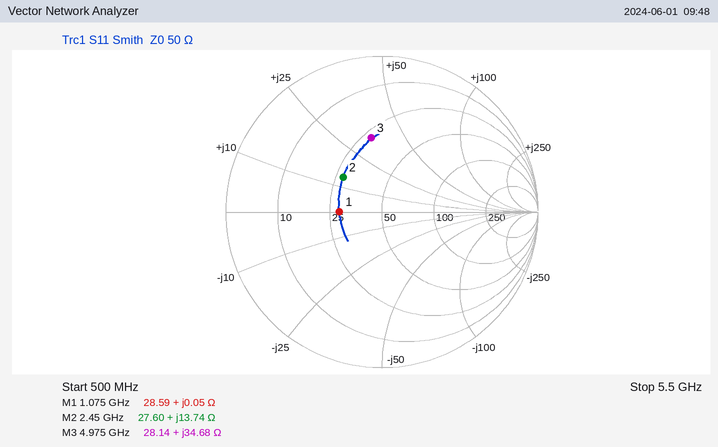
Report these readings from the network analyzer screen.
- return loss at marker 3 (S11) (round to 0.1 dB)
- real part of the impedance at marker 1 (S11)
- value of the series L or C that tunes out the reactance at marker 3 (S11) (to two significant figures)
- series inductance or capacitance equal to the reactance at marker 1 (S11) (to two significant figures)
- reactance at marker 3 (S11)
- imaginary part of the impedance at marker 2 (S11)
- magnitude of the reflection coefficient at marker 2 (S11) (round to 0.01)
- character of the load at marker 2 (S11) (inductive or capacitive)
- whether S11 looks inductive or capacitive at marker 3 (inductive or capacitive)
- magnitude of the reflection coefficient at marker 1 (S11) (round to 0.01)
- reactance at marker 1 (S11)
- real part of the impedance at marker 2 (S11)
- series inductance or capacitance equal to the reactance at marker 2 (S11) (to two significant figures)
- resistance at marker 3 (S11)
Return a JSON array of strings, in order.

["6.4 dB", "28.59 Ω", "920 fF", "7.4 pH", "+34.68 Ω", "+13.74 Ω", "0.33", "inductive", "inductive", "0.27", "+0.05 Ω", "27.60 Ω", "890 pH", "28.14 Ω"]
